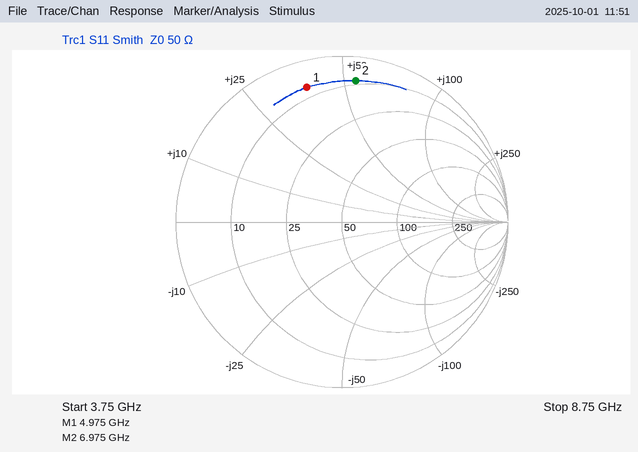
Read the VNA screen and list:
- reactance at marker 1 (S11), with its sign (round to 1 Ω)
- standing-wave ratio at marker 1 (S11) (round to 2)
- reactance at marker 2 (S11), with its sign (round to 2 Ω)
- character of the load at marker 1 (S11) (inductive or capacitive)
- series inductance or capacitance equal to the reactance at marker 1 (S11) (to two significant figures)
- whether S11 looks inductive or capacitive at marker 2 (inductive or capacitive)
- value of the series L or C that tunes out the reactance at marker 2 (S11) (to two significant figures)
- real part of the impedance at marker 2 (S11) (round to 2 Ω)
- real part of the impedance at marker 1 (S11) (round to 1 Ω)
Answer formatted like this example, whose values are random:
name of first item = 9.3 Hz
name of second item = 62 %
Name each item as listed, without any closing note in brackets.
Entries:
reactance at marker 1 (S11), with its sign = +38 Ω
standing-wave ratio at marker 1 (S11) = 12
reactance at marker 2 (S11), with its sign = +54 Ω
character of the load at marker 1 (S11) = inductive
series inductance or capacitance equal to the reactance at marker 1 (S11) = 1.2 nH
whether S11 looks inductive or capacitive at marker 2 = inductive
value of the series L or C that tunes out the reactance at marker 2 (S11) = 420 fF
real part of the impedance at marker 2 (S11) = 8 Ω
real part of the impedance at marker 1 (S11) = 7 Ω
